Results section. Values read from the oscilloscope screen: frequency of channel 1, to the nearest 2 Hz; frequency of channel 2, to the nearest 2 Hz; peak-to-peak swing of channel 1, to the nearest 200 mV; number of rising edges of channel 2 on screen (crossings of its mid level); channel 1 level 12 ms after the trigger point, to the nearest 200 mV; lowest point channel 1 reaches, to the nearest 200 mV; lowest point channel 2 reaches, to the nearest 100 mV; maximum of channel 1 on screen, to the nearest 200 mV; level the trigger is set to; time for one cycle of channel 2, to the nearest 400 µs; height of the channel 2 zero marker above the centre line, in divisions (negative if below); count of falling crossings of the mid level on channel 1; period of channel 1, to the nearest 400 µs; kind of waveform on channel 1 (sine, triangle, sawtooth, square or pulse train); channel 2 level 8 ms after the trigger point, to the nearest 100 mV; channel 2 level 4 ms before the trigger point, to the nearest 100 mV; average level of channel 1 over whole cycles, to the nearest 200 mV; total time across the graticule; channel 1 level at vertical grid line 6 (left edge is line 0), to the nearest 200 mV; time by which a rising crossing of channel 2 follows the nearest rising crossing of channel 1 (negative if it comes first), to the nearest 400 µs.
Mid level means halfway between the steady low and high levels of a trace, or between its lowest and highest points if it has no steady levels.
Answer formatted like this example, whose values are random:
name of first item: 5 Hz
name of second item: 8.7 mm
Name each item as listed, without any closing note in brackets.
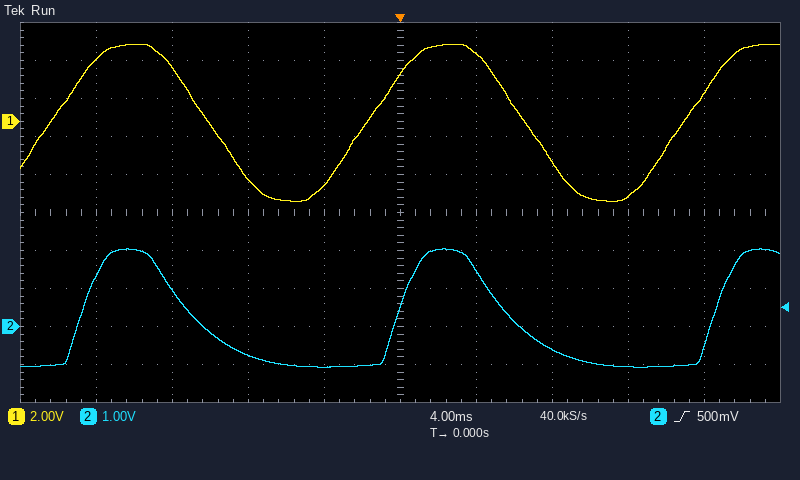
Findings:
frequency of channel 1, to the nearest 2 Hz: 60 Hz
frequency of channel 2, to the nearest 2 Hz: 60 Hz
peak-to-peak swing of channel 1, to the nearest 200 mV: 8.2 V
number of rising edges of channel 2 on screen: 3
channel 1 level 12 ms after the trigger point, to the nearest 200 mV: -4.0 V
lowest point channel 1 reaches, to the nearest 200 mV: -4.2 V
lowest point channel 2 reaches, to the nearest 100 mV: -1.1 V
maximum of channel 1 on screen, to the nearest 200 mV: 4.0 V
level the trigger is set to: 500 mV
time for one cycle of channel 2, to the nearest 400 µs: 16.8 ms
height of the channel 2 zero marker above the centre line, in divisions: -3.0 div
count of falling crossings of the mid level on channel 1: 2
period of channel 1, to the nearest 400 µs: 16.8 ms
kind of waveform on channel 1: sine
channel 2 level 8 ms after the trigger point, to the nearest 100 mV: -600 mV
channel 2 level 4 ms before the trigger point, to the nearest 100 mV: -1.1 V
average level of channel 1 over whole cycles, to the nearest 200 mV: 0.0 V
total time across the graticule: 40 ms
channel 1 level at vertical grid line 6 (left edge is line 0), to the nearest 200 mV: 3.6 V
time by which a rising crossing of channel 2 follows the nearest rising crossing of channel 1 (negative if it comes first), to the nearest 400 µs: +1.6 ms
